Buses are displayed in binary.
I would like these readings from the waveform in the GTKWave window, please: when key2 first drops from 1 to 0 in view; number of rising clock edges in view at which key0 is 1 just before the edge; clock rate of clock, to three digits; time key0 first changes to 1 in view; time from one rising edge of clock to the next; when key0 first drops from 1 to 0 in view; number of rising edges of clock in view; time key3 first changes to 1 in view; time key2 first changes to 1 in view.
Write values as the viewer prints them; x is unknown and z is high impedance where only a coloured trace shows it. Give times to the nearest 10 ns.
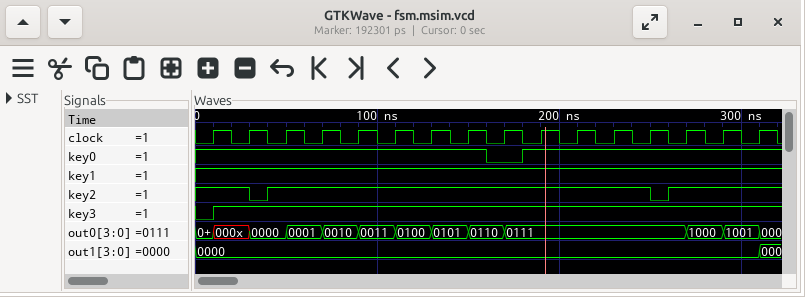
30 ns
15
50.0 MHz
180 ns
20 ns
160 ns
16
10 ns
40 ns
